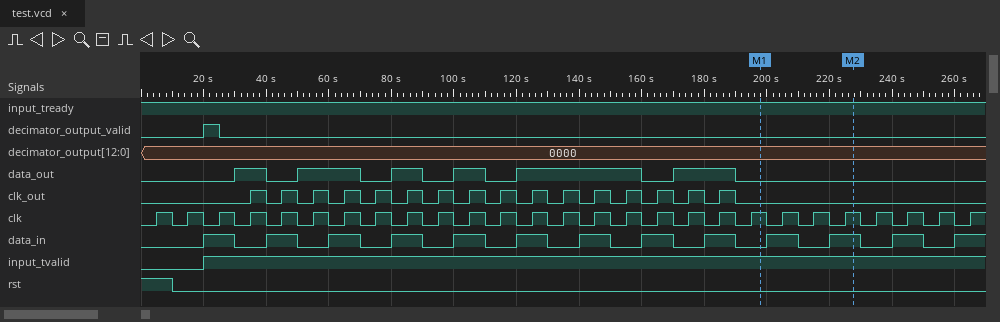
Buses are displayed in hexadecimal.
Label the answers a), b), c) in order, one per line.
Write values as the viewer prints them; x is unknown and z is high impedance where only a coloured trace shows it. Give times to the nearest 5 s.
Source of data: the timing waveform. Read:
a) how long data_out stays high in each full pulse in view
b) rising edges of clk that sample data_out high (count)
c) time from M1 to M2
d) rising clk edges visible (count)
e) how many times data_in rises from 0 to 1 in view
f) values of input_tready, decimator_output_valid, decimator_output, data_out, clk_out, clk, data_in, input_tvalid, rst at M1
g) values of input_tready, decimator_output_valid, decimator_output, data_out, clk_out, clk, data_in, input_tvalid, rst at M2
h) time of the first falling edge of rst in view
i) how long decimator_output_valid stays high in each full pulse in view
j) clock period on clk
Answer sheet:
a) 10 s, 20 s, 10 s, 10 s, 40 s, 20 s
b) 11
c) 30 s
d) 27
e) 13
f) input_tready=1, decimator_output_valid=0, decimator_output=0000, data_out=0, clk_out=0, clk=1, data_in=0, input_tvalid=1, rst=0
g) input_tready=1, decimator_output_valid=0, decimator_output=0000, data_out=0, clk_out=0, clk=1, data_in=1, input_tvalid=1, rst=0
h) 10 s
i) 5 s
j) 10 s
